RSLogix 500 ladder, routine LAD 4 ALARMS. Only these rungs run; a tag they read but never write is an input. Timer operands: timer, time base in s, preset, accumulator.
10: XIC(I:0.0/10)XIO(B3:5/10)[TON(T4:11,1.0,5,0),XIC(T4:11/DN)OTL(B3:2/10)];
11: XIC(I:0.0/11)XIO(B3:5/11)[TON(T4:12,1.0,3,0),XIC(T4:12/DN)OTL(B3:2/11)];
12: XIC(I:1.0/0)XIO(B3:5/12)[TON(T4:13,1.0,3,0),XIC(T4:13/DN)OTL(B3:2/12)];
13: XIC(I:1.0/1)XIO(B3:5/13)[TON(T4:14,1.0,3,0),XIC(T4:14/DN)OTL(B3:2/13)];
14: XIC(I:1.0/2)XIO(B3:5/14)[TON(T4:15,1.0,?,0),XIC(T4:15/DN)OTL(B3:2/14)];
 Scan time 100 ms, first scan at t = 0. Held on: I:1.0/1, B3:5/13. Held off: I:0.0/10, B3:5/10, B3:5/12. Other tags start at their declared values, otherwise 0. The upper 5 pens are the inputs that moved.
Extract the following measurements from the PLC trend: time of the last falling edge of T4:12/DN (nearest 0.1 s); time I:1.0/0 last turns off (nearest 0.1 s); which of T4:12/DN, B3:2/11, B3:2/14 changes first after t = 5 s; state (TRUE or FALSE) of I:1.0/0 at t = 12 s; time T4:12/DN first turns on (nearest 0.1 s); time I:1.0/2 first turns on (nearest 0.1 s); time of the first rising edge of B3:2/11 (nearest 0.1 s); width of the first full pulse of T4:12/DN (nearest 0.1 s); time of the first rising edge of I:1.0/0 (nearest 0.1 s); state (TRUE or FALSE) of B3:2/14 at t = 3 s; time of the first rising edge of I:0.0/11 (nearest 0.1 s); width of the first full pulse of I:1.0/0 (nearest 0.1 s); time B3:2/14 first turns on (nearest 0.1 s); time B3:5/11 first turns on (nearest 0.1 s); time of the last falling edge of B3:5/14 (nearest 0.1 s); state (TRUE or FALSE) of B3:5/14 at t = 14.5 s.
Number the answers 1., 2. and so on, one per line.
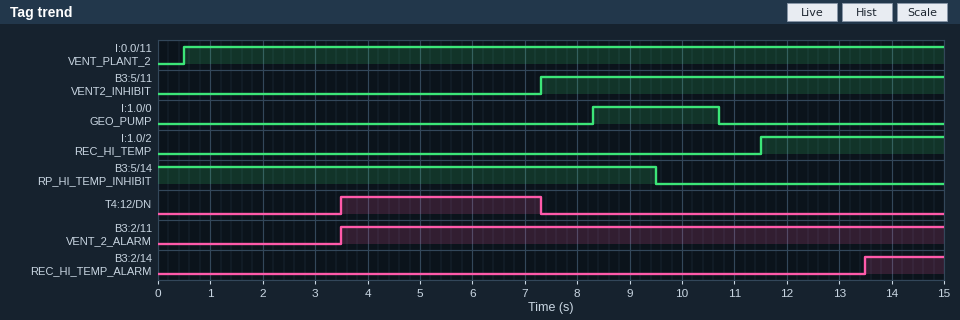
1. 7.3 s
2. 10.7 s
3. T4:12/DN
4. FALSE
5. 3.5 s
6. 11.5 s
7. 3.5 s
8. 3.8 s
9. 8.3 s
10. FALSE
11. 0.5 s
12. 2.4 s
13. 13.5 s
14. 7.3 s
15. 9.5 s
16. FALSE
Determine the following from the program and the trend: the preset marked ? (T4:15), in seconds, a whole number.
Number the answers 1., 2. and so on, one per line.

1. 2 s
